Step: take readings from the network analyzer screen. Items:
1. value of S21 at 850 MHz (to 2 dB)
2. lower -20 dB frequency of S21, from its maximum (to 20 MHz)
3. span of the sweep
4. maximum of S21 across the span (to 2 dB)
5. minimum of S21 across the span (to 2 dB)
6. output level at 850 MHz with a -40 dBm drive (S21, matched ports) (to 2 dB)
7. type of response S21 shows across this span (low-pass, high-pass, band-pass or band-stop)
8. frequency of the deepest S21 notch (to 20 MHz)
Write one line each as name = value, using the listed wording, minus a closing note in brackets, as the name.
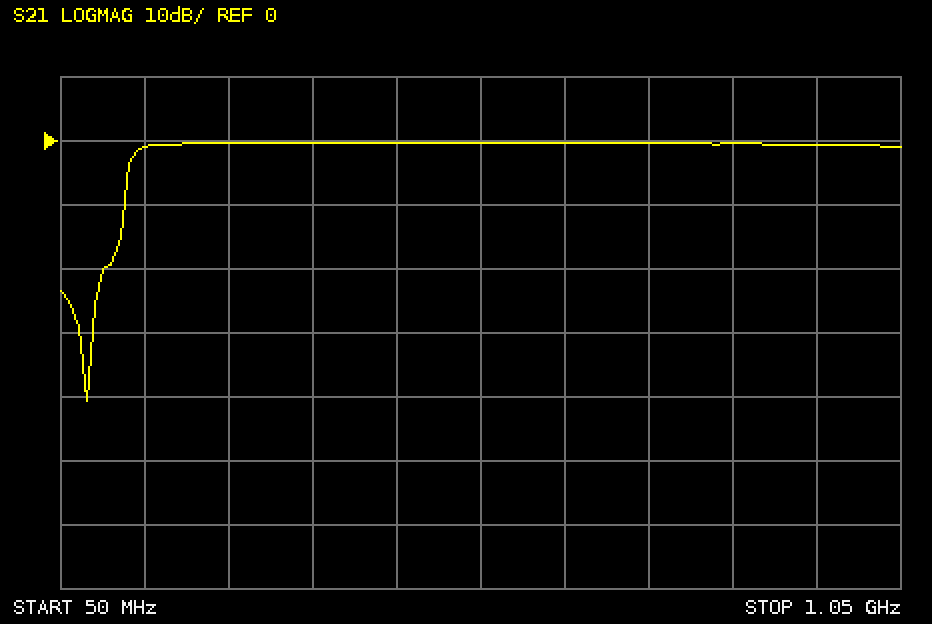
value of S21 at 850 MHz = 0 dB
lower -20 dB frequency of S21, from its maximum = 100 MHz
span of the sweep = 1 GHz
maximum of S21 across the span = 0 dB
minimum of S21 across the span = -40 dB
output level at 850 MHz with a -40 dBm drive (S21, matched ports) = -40 dBm
type of response S21 shows across this span = high-pass
frequency of the deepest S21 notch = 80 MHz
